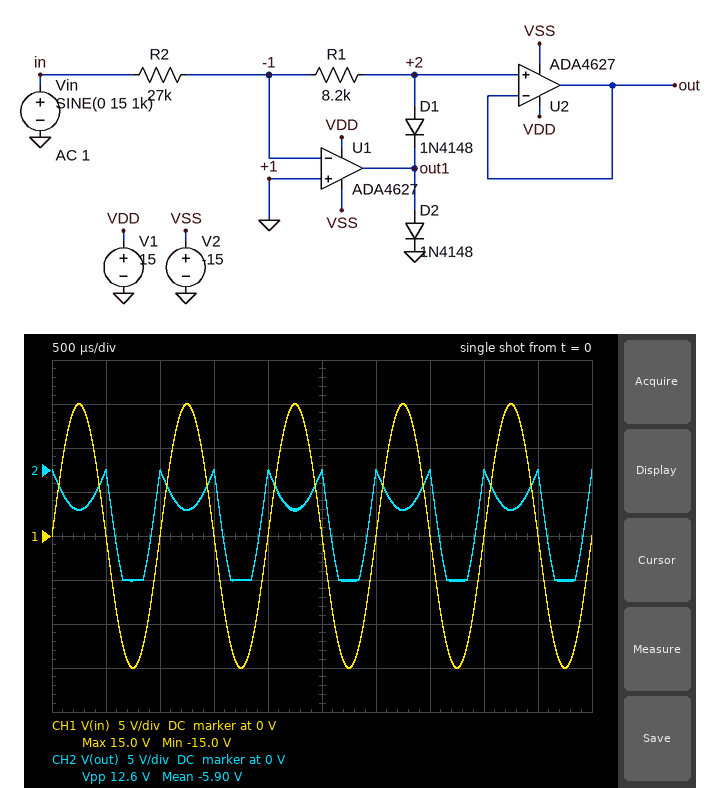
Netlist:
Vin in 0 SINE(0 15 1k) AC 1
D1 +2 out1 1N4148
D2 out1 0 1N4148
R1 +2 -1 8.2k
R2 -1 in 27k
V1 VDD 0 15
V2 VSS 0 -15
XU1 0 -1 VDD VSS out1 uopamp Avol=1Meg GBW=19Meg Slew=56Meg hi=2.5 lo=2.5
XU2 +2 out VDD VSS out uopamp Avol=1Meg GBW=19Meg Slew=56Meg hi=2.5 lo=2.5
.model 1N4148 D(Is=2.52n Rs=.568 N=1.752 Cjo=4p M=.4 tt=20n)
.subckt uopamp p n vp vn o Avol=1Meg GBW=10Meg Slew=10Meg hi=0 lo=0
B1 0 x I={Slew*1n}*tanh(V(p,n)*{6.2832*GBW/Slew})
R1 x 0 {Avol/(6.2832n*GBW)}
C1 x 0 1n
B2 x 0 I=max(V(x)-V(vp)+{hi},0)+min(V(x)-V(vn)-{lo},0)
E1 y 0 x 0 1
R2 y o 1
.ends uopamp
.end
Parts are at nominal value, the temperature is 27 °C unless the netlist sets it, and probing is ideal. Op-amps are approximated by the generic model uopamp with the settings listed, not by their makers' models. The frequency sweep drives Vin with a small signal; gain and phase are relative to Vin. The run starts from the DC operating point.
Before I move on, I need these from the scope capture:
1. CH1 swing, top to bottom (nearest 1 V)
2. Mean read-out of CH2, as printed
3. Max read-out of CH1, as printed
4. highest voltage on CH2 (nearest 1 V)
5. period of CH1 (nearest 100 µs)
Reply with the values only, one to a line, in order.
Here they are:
30 V
-5.90 V
15.0 V
0 V
1.0 ms
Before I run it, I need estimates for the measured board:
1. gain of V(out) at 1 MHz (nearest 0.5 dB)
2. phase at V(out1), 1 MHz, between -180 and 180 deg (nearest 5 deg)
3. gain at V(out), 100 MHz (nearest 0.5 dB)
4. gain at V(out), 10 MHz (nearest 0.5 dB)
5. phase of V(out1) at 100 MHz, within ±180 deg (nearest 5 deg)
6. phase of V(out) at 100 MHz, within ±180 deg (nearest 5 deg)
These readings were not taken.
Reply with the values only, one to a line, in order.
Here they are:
-13.5 dB
100 deg
-44.5 dB
-16.0 dB
95 deg
20 deg
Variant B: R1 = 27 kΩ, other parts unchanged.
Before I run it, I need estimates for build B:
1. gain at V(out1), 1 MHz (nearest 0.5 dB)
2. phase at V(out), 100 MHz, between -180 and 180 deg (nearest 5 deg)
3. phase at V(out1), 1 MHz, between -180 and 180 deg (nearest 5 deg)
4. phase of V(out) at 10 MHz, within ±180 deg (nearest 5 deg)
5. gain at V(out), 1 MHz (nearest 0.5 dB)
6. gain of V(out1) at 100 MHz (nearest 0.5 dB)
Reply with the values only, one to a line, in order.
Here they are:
4.5 dB
15 deg
120 deg
110 deg
-1.5 dB
-20.5 dB
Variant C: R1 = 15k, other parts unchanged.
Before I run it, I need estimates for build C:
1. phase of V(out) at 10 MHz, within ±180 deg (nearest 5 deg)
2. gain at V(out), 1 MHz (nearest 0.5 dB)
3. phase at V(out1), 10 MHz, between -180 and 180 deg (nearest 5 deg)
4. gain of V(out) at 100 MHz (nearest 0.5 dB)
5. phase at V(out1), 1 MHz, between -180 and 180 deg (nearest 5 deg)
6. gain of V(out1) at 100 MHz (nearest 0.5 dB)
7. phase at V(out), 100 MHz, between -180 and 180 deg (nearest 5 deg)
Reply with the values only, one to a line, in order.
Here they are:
115 deg
-7.0 dB
130 deg
-39.5 dB
105 deg
-23.5 dB
20 deg
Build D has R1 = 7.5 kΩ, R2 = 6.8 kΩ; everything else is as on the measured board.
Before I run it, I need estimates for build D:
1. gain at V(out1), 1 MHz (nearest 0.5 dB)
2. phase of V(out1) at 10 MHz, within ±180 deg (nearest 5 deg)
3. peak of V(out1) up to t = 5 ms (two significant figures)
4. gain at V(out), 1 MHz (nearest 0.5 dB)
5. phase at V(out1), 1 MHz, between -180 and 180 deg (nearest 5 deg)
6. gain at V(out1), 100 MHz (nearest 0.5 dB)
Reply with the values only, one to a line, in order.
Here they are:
13.0 dB
110 deg
5.2 V
-4.5 dB
95 deg
-20.0 dB
